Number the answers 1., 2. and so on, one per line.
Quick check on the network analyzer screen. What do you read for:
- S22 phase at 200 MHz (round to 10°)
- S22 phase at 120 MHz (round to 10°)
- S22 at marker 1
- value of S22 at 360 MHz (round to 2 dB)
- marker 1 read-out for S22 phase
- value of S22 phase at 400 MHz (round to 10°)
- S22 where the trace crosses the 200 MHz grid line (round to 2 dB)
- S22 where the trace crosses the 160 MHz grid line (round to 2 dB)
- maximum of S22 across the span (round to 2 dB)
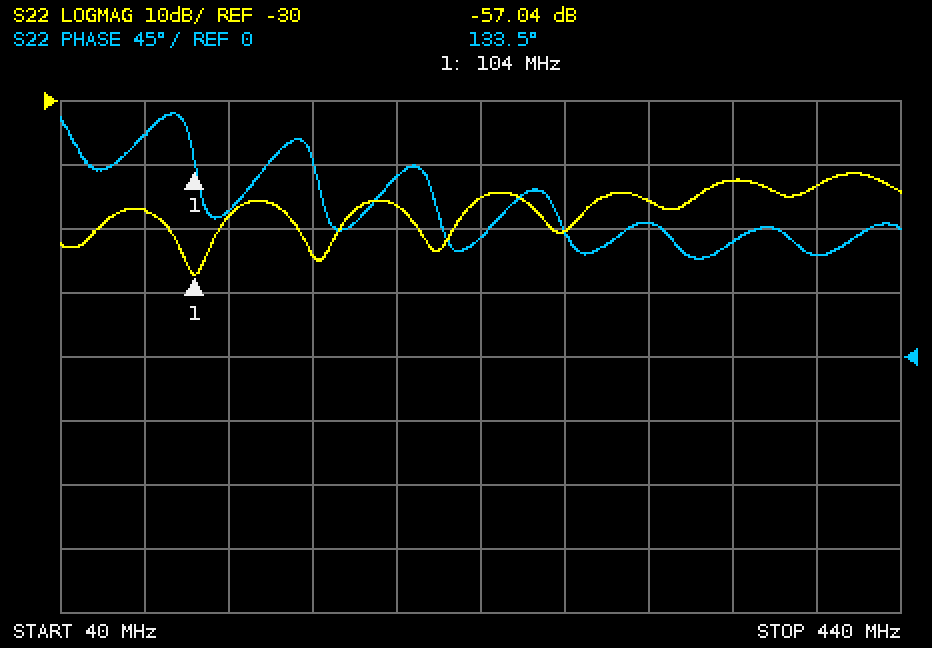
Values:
1. 130°
2. 100°
3. -57.04 dB
4. -42 dB
5. 133.5°
6. 70°
7. -46 dB
8. -54 dB
9. -42 dB
